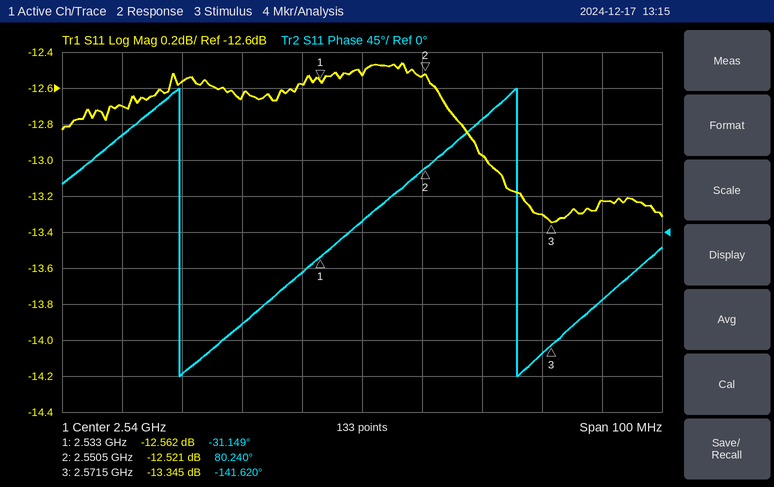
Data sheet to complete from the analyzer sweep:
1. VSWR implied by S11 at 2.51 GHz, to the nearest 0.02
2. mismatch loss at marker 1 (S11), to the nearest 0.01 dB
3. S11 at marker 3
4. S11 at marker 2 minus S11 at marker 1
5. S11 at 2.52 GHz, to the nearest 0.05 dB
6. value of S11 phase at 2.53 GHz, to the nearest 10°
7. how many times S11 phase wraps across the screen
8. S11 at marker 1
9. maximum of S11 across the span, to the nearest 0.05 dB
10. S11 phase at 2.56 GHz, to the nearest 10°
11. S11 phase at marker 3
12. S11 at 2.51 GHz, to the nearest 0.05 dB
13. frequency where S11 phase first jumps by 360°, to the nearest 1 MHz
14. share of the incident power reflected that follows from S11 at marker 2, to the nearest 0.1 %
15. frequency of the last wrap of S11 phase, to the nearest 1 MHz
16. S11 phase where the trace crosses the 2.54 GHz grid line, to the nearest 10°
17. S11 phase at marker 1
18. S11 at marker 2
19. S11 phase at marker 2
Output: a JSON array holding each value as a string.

["1.62", "0.25 dB", "-13.345 dB", "0.041 dB", "-12.65 dB", "-50°", "2", "-12.562 dB", "-12.45 dB", "140°", "-141.620°", "-12.55 dB", "2.510 GHz", "5.6 %", "2.566 GHz", "10°", "-31.149°", "-12.521 dB", "80.240°"]
